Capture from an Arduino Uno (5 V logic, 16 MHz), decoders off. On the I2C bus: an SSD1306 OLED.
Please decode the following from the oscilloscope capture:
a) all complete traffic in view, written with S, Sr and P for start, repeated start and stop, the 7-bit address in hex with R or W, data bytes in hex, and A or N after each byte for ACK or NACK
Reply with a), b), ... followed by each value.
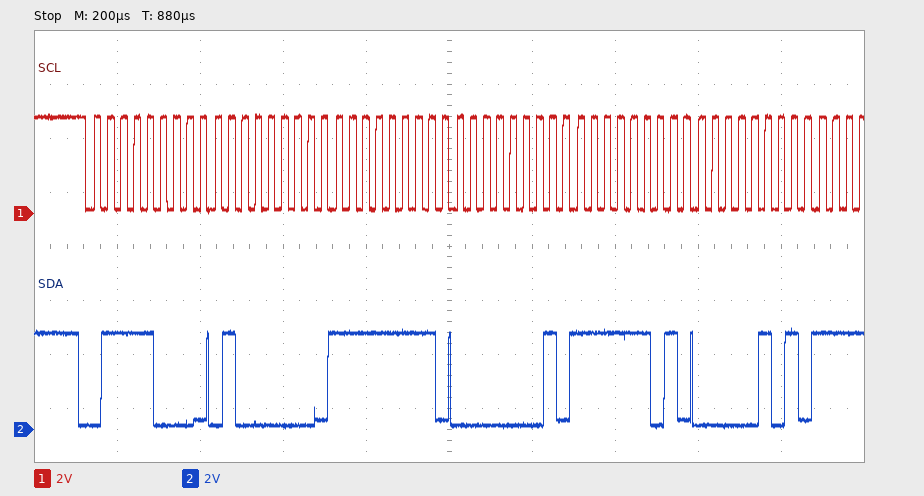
a) S 3CW A 40 A FF A 01 A FD A 05 A
